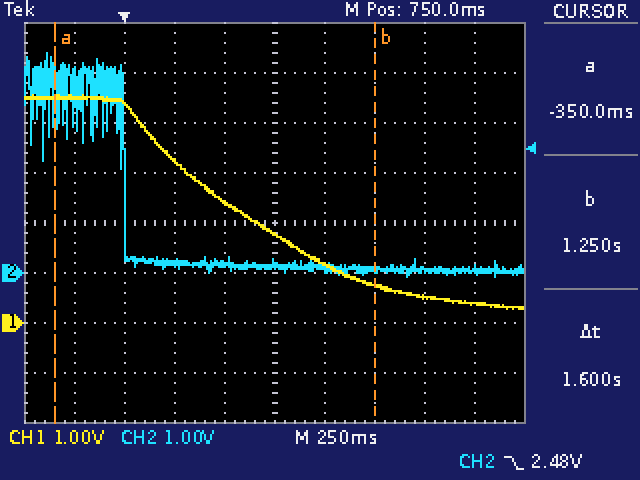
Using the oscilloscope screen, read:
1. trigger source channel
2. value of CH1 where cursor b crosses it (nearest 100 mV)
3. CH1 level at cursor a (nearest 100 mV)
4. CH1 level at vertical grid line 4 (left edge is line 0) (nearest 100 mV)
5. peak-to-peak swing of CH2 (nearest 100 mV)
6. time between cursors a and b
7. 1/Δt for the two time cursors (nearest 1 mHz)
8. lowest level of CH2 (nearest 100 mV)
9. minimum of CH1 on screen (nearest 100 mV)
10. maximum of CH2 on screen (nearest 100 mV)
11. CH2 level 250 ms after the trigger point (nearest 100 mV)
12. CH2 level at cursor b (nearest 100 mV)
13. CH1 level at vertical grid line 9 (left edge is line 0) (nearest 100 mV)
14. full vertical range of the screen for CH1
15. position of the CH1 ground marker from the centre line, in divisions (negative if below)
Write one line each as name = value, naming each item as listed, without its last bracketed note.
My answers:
trigger source channel = CH2
value of CH1 where cursor b crosses it = 700 mV
CH1 level at cursor a = 4.5 V
CH1 level at vertical grid line 4 (left edge is line 0) = 2.4 V
peak-to-peak swing of CH2 = 4.5 V
time between cursors a and b = 1.6 s
1/Δt for the two time cursors = 625 mHz
lowest level of CH2 = -100 mV
minimum of CH1 on screen = 300 mV
maximum of CH2 on screen = 4.4 V
CH2 level 250 ms after the trigger point = 200 mV
CH2 level at cursor b = 100 mV
CH1 level at vertical grid line 9 (left edge is line 0) = 400 mV
full vertical range of the screen for CH1 = 8 V
position of the CH1 ground marker from the centre line, in divisions = -2.0 div
